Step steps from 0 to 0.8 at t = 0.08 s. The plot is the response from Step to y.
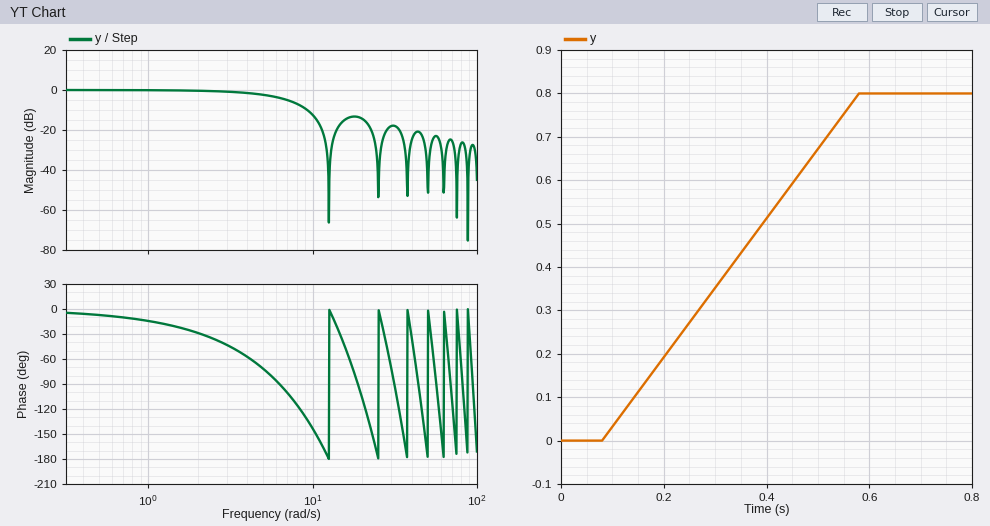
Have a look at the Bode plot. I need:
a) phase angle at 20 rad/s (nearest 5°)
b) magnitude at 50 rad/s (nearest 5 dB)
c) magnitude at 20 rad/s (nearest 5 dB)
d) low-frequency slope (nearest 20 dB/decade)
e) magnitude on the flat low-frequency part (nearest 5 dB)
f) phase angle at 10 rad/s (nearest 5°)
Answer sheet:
-105°
-45 dB
-15 dB
0 dB/decade
0 dB
-145°
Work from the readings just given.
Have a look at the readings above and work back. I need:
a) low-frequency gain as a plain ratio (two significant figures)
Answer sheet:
1.0
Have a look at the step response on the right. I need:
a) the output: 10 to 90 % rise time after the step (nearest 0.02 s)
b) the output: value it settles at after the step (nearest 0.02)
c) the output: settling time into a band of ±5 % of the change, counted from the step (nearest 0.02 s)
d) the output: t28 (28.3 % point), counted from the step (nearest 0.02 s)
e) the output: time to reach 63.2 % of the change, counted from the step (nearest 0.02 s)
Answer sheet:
0.40 s
0.80
0.48 s
0.14 s
0.32 s
